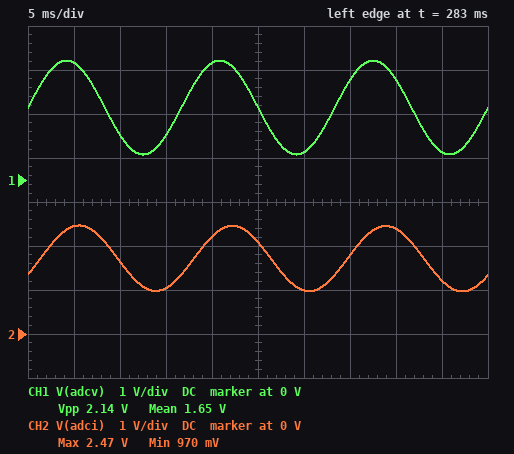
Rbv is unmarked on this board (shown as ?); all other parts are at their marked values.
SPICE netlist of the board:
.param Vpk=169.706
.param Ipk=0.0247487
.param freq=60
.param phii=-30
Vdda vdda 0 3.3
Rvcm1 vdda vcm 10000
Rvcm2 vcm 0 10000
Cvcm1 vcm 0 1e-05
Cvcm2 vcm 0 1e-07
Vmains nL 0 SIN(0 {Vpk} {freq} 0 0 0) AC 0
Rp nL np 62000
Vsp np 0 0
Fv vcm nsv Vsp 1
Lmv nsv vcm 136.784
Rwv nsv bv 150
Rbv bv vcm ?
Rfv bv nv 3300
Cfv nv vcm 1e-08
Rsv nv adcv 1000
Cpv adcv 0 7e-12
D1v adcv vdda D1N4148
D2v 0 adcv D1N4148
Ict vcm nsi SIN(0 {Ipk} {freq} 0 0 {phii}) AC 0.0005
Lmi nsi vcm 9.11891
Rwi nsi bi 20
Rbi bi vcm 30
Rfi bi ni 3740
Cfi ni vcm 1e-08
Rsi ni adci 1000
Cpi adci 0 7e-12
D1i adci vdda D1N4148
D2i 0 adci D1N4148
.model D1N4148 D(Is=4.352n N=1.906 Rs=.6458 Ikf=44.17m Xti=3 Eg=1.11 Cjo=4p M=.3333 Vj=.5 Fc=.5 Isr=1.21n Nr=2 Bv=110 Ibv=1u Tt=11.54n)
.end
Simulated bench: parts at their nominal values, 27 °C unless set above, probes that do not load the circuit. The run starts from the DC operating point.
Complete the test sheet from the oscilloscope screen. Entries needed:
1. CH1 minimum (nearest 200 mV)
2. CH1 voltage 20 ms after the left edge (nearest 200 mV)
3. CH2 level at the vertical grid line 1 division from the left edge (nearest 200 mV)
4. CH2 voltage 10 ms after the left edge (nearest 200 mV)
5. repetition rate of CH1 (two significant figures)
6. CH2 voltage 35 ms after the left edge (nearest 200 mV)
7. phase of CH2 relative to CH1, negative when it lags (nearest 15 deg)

600 mV
2.6 V
2.4 V
1.6 V
60 Hz
1.8 V
-30 deg
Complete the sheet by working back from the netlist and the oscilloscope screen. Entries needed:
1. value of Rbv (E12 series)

390 Ω
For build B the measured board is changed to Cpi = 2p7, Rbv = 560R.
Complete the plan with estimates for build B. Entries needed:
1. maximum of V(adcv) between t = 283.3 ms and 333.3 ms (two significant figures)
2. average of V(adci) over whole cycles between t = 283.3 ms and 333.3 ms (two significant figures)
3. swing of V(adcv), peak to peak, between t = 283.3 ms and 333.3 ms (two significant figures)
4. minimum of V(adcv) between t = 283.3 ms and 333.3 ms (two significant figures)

3.2 V
1.7 V
3.1 V
110 mV
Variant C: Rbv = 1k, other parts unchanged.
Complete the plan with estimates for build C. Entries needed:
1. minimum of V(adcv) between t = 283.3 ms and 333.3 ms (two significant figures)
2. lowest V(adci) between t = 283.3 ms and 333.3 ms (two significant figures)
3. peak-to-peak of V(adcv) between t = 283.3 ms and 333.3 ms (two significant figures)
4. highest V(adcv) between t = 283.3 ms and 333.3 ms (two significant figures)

-500 mV
980 mV
4.3 V
3.8 V
